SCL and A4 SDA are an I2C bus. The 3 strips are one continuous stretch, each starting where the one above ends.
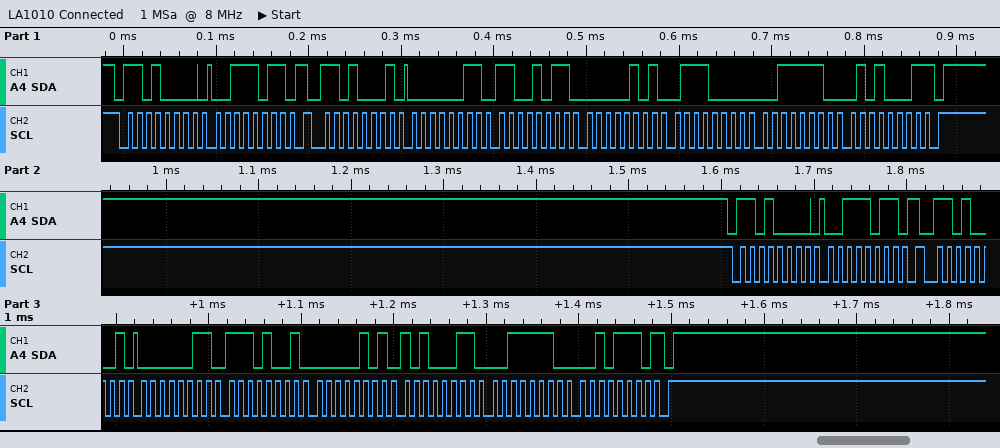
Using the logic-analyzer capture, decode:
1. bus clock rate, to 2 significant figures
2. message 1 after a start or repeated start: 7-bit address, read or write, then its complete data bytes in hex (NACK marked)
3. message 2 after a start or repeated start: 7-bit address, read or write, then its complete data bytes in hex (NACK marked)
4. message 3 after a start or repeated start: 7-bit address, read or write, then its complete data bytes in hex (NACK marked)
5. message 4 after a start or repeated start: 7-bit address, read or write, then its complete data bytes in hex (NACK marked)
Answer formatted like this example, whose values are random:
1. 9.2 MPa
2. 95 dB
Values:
1. 100 kHz
2. 0x68 write: 3B
3. 0x68 read: 03 CB 05 70 3E 51 NACK
4. 0x68 write: 3B
5. 0x68 read: 03 E9 05 A3 3E 2E NACK
